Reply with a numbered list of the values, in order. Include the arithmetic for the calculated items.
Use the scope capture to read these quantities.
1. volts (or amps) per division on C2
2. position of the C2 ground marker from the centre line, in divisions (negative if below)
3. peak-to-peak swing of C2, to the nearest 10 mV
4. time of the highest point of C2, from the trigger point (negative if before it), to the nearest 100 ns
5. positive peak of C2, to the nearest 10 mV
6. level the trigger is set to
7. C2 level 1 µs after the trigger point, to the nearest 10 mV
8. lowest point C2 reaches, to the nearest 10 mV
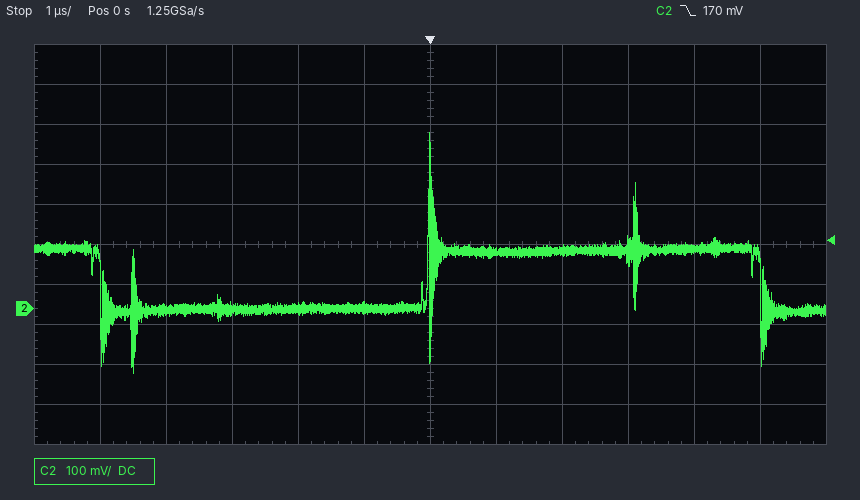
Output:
1. 100 mV
2. -1.6 div
3. 440 mV − (-160 mV) = 600 mV
4. 0.0 µs
5. 440 mV
6. 170 mV
7. 140 mV
8. -160 mV
